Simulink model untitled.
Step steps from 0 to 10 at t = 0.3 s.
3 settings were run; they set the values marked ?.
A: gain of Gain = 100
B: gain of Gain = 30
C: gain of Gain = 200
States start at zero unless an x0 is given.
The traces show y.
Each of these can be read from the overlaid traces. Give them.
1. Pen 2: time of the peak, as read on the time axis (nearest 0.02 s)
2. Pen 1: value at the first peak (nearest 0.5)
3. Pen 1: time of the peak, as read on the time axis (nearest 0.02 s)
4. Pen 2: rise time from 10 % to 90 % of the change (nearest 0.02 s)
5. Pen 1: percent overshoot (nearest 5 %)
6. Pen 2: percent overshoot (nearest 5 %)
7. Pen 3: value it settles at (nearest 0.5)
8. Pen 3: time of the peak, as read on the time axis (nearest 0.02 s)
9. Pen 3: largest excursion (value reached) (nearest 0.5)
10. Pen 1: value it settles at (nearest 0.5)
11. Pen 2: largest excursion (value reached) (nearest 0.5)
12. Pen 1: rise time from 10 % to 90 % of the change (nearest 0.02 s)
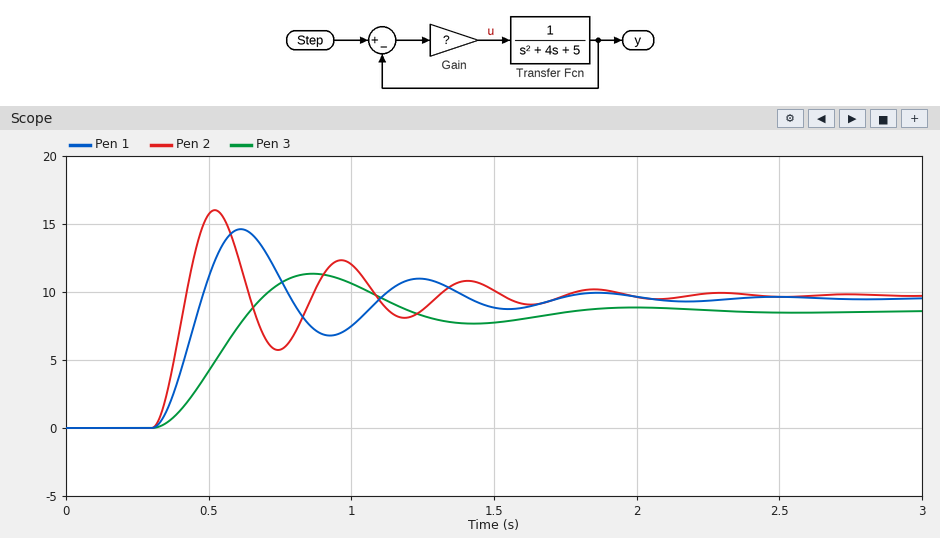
0.52 s
14.5
0.62 s
0.08 s
55 %
65 %
8.5
0.86 s
11.5
9.5
16.0
0.12 s
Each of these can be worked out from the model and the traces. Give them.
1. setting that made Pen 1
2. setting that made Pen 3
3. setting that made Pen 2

A
B
C
